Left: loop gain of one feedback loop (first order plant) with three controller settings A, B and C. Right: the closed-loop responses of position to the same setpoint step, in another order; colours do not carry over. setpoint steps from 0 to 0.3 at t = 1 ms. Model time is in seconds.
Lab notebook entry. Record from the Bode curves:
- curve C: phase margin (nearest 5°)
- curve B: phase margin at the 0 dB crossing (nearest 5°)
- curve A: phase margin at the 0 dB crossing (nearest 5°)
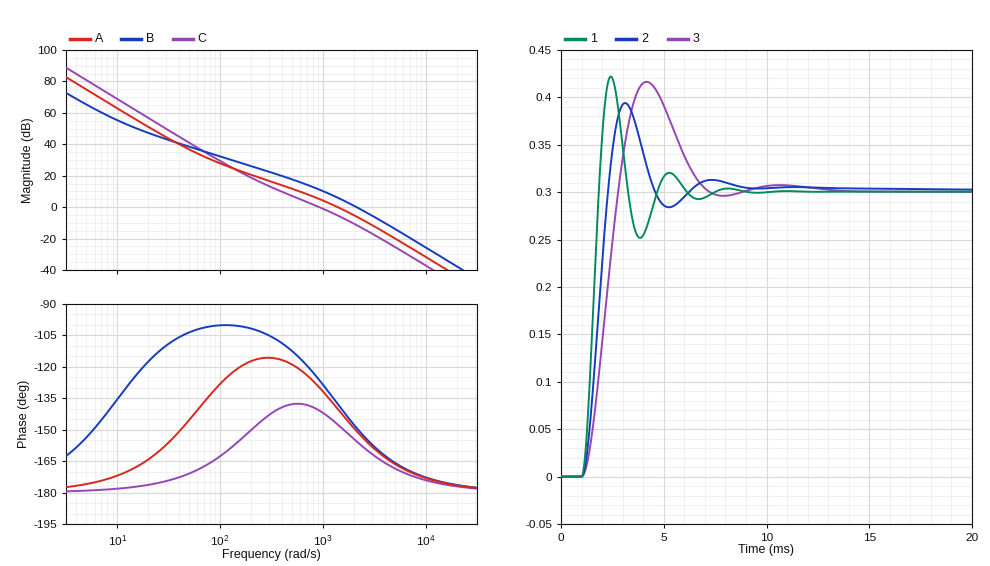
40°
30°
40°
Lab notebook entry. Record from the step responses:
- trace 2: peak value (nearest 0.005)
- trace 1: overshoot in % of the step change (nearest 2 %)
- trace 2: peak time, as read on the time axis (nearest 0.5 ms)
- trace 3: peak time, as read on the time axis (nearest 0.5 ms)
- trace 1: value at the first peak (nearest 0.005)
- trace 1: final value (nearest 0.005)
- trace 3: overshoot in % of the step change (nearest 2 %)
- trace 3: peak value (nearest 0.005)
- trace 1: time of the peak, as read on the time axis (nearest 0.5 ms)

0.395
40 %
3.0 ms
4.0 ms
0.420
0.300
38 %
0.415
2.5 ms
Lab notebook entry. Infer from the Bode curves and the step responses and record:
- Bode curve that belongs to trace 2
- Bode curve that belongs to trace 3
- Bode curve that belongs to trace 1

A
C
B
